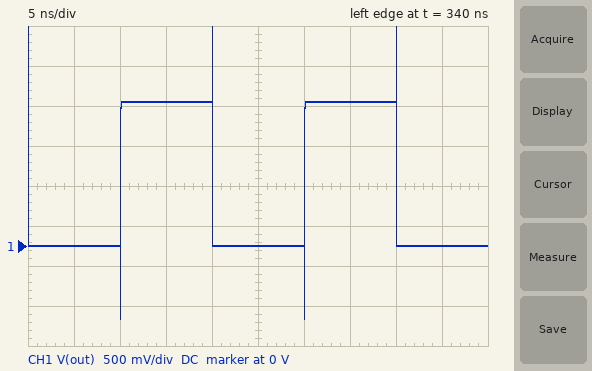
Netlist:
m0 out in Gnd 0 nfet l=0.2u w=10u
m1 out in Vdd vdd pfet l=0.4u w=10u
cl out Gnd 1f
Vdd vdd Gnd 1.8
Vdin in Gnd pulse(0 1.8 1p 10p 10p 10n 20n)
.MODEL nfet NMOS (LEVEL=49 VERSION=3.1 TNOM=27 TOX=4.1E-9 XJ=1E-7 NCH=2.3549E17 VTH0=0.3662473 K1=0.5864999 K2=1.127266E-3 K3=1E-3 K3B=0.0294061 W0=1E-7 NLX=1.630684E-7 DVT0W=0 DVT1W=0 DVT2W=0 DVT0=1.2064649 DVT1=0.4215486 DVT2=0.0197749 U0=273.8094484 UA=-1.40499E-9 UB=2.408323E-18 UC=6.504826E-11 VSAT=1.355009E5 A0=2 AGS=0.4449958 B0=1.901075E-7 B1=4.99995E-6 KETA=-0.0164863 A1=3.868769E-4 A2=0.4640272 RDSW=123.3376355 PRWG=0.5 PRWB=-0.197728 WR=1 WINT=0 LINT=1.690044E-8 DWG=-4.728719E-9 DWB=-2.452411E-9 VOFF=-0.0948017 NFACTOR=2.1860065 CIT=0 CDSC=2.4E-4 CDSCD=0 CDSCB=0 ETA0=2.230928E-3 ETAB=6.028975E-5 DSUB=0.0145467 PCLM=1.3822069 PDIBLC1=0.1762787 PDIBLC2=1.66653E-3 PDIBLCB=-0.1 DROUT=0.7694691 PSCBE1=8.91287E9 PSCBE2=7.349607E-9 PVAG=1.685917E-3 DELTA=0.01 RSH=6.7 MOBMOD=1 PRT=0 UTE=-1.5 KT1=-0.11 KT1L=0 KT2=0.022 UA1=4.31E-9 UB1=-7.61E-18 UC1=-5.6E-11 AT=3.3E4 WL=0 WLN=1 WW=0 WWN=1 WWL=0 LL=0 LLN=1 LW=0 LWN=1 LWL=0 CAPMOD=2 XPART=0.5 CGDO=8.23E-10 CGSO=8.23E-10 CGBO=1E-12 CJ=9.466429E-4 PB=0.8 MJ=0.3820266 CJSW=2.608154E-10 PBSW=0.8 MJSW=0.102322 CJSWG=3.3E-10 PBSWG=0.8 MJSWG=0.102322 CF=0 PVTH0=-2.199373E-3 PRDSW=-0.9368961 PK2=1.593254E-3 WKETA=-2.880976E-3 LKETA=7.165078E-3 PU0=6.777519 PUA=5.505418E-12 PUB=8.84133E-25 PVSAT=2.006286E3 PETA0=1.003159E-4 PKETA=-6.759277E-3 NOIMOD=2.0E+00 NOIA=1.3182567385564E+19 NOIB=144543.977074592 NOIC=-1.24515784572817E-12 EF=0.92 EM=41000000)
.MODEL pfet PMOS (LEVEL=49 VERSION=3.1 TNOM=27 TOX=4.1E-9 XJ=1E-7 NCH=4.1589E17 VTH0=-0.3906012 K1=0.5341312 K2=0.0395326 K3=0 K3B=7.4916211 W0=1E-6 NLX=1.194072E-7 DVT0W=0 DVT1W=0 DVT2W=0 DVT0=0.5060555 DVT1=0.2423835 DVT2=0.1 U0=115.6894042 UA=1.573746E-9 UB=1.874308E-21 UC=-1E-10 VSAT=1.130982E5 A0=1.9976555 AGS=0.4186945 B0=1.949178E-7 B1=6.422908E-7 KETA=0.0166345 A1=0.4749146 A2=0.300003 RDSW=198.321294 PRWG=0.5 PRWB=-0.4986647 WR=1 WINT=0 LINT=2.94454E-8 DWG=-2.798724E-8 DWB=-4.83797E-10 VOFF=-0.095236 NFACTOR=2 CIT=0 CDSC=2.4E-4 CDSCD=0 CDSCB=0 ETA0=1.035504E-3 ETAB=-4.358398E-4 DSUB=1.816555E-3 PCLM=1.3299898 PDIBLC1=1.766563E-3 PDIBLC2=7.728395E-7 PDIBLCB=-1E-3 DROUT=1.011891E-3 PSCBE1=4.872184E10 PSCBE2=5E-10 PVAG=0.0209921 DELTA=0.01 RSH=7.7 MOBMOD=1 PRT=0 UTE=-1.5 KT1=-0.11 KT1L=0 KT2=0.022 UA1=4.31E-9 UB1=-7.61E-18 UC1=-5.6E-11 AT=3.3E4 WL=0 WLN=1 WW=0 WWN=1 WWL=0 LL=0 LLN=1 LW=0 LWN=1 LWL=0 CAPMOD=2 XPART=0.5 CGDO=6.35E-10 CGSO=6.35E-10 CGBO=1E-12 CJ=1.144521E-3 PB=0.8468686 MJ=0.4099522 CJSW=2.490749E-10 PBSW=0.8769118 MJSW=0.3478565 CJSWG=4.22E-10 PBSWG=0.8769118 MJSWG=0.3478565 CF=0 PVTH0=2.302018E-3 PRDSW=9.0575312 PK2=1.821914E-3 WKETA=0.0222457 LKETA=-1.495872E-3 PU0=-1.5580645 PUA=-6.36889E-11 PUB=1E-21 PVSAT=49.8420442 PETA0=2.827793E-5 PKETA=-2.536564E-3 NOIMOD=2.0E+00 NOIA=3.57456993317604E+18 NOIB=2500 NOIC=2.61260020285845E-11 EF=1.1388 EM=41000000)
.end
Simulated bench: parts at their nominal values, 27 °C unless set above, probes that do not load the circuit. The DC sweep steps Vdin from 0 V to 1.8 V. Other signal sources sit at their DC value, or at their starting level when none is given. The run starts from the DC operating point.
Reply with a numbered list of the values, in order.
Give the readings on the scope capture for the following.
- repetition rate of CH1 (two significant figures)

1. 50 MHz
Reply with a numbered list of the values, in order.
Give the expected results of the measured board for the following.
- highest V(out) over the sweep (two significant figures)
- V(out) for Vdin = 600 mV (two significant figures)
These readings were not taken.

1. 1.8 V
2. 1.7 V
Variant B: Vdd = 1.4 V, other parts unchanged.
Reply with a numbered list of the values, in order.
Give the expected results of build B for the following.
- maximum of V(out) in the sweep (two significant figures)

1. 1.4 V
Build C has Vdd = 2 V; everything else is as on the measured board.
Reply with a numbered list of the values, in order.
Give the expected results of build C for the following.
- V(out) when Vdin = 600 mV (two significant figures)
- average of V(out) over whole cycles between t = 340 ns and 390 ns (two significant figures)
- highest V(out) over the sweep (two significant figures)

1. 1.9 V
2. 1.0 V
3. 2.0 V
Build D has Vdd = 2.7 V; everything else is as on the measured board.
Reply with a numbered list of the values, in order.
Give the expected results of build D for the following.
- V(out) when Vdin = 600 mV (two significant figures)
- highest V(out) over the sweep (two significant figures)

1. 2.6 V
2. 2.7 V
